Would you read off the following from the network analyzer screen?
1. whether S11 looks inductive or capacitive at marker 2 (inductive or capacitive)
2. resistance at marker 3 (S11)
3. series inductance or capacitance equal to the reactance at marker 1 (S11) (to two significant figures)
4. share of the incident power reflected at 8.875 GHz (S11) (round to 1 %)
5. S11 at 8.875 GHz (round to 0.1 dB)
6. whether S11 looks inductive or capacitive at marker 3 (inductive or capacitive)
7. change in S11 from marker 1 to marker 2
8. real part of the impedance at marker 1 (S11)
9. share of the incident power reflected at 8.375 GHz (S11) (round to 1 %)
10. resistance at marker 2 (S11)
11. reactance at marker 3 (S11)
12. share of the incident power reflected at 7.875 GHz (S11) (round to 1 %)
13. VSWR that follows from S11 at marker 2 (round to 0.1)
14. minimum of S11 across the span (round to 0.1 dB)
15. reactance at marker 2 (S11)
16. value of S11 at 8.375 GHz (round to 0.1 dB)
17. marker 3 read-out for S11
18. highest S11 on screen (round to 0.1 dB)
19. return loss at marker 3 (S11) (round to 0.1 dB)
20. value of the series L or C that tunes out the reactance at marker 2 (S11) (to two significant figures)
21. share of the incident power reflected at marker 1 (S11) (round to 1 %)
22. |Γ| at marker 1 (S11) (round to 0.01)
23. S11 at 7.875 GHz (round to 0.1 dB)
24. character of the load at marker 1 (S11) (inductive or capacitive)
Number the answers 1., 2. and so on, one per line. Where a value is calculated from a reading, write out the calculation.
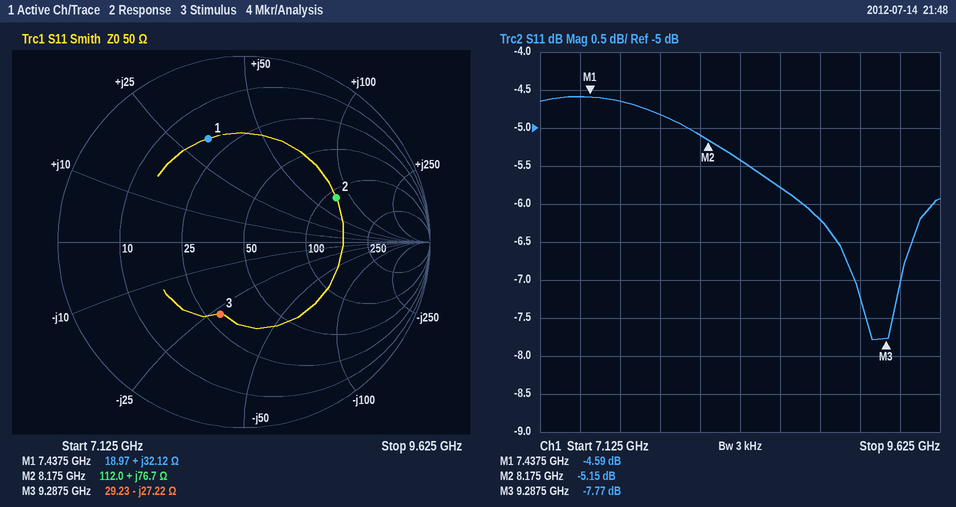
1. inductive
2. 29.23 Ω
3. L = 32.12 Ω/(2π × 7.4375 GHz) ≈ 687 pH, so 690 pH to two significant figures
4. 10^(-6.2/10) ≈ 24 %
5. -6.2 dB
6. capacitive
7. -5.15 − (-4.59) = -0.56 dB
8. 18.97 Ω
9. 10^(-5.4/10) ≈ 29 %
10. 112.0 Ω
11. -27.22 Ω
12. 10^(-4.8/10) ≈ 33 %
13. (1 + 0.5527)/(1 − 0.5527) ≈ 3.5
14. -7.8 dB
15. +76.7 Ω
16. -5.4 dB
17. -7.77 dB
18. -4.6 dB
19. 7.8 dB
20. C = 1/(2π × 8.175 GHz × 76.7 Ω) ≈ 254 fF, so 250 fF to two significant figures
21. 10^(-4.59/10) ≈ 35 %
22. 0.59
23. -4.8 dB
24. inductive
